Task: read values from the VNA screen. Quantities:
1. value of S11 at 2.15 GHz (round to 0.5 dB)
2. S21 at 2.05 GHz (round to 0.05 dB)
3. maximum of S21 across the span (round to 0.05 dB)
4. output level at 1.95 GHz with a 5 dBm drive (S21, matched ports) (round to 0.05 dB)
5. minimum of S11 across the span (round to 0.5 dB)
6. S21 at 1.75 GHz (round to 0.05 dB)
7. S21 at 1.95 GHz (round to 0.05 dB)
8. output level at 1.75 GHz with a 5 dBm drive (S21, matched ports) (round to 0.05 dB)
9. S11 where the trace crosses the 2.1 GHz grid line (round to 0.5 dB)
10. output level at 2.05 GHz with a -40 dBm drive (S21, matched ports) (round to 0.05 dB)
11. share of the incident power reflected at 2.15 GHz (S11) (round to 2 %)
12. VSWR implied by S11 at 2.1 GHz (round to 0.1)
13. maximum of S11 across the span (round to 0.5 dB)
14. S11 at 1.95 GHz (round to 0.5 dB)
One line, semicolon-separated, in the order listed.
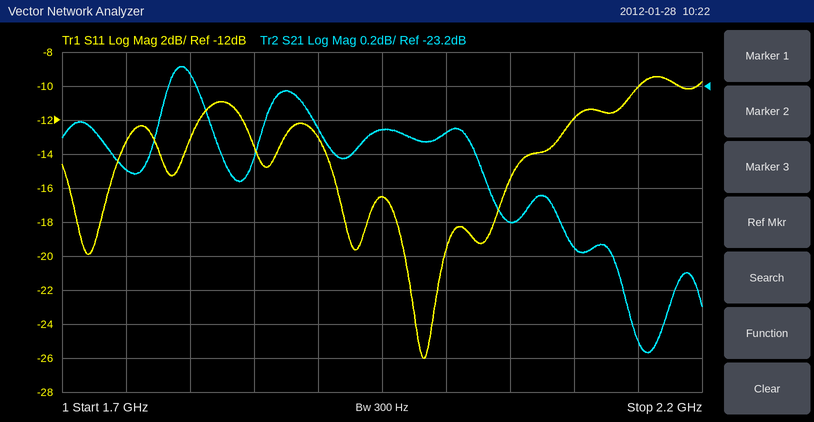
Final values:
-10.0 dB; -24.00 dB; -23.10 dB; -18.45 dBm; -26.0 dB; -23.70 dB; -23.45 dB; -18.70 dBm; -12.0 dB; -64.00 dBm; 10 %; 1.7; -9.5 dB; -16.5 dB
